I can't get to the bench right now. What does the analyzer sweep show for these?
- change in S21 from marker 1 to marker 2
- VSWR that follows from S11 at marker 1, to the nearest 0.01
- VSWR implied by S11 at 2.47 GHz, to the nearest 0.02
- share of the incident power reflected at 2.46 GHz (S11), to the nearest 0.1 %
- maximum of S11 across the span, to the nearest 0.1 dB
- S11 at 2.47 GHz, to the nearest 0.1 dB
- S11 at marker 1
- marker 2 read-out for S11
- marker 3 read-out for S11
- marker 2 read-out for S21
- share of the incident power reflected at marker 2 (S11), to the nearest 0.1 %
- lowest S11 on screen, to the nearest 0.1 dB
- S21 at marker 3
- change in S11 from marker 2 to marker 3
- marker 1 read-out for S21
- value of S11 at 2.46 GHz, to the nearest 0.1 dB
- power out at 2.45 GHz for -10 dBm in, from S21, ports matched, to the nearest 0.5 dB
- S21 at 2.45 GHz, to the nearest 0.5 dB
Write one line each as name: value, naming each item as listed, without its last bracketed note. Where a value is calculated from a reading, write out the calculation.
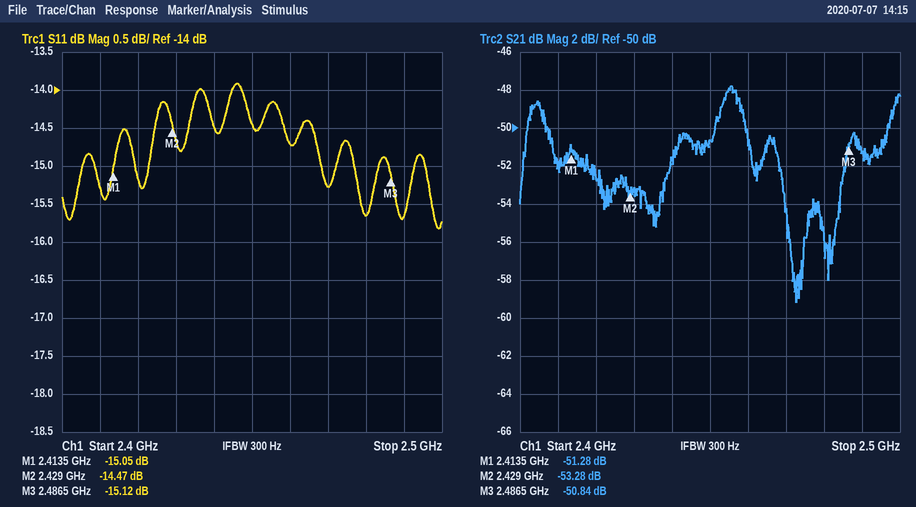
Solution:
change in S21 from marker 1 to marker 2: -53.28 − (-51.28) = -2.00 dB
VSWR that follows from S11 at marker 1, to the nearest 0.01: (1 + 0.1768)/(1 − 0.1768) ≈ 1.43
VSWR implied by S11 at 2.47 GHz, to the nearest 0.02: |Γ| = 10^(-15.3/20) = 0.1718; VSWR = (1 + 0.1718)/(1 − 0.1718) ≈ 1.41, so 1.42 to the nearest 0.02
share of the incident power reflected at 2.46 GHz (S11), to the nearest 0.1 %: 10^(-14.7/10) ≈ 3.4 %
maximum of S11 across the span, to the nearest 0.1 dB: -13.9 dB
S11 at 2.47 GHz, to the nearest 0.1 dB: -15.3 dB
S11 at marker 1: -15.05 dB
marker 2 read-out for S11: -14.47 dB
marker 3 read-out for S11: -15.12 dB
marker 2 read-out for S21: -53.28 dB
share of the incident power reflected at marker 2 (S11), to the nearest 0.1 %: 10^(-14.47/10) ≈ 3.6 %
lowest S11 on screen, to the nearest 0.1 dB: -15.8 dB
S21 at marker 3: -50.84 dB
change in S11 from marker 2 to marker 3: -15.12 − (-14.47) = -0.65 dB
marker 1 read-out for S21: -51.28 dB
value of S11 at 2.46 GHz, to the nearest 0.1 dB: -14.7 dB
power out at 2.45 GHz for -10 dBm in, from S21, ports matched, to the nearest 0.5 dB: -10 dBm + (-50.5 dB) = -60.5 dBm
S21 at 2.45 GHz, to the nearest 0.5 dB: -50.5 dB
